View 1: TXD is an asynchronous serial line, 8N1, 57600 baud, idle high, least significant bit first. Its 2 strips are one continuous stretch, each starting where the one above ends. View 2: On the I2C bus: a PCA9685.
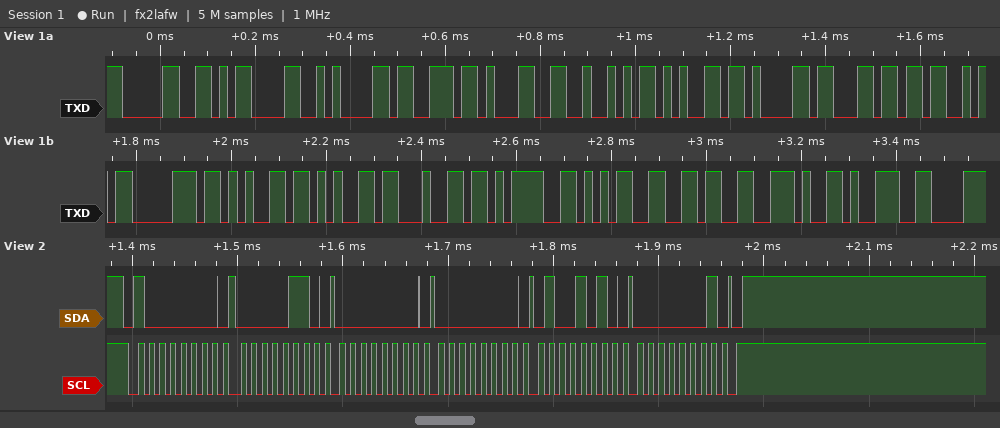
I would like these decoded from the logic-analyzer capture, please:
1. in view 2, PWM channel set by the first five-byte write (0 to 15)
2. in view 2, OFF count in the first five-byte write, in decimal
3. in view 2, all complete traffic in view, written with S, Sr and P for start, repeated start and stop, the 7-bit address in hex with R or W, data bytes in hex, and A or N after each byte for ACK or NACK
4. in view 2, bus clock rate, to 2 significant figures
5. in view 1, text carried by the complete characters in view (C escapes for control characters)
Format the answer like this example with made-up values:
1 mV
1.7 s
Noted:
0
330
S 40W A 06 A 00 A 00 A 4A A 01 A P
100 kHz
"0\r\ns1RealSpeed=56.9"
